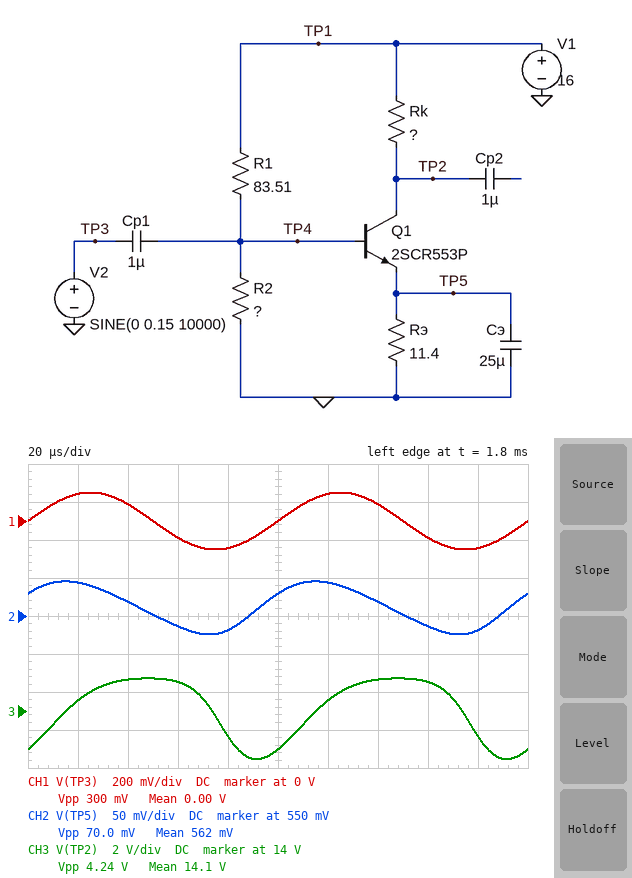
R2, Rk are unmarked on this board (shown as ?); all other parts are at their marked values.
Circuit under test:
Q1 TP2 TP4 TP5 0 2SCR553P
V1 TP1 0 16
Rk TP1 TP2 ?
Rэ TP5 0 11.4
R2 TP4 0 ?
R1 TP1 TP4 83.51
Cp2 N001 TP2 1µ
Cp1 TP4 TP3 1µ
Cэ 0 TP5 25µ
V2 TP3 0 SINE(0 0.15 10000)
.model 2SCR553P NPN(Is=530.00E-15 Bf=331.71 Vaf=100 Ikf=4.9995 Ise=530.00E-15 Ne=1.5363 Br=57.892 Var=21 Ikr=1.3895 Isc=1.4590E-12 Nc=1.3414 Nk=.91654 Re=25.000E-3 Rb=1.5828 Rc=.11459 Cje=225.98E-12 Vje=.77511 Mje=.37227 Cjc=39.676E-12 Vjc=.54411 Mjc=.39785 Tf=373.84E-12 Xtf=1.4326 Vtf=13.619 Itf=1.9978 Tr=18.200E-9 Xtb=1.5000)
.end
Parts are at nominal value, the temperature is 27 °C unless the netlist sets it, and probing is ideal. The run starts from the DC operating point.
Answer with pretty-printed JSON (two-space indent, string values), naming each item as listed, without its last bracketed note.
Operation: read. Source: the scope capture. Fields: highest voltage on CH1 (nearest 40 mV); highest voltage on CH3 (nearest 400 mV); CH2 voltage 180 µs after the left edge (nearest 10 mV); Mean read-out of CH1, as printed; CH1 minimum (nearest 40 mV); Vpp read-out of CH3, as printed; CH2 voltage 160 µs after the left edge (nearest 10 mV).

{
  "highest voltage on CH1": "160 mV",
  "highest voltage on CH3": "15.6 V",
  "CH2 voltage 180 µs after the left edge": "530 mV",
  "Mean read-out of CH1, as printed": "0.00 V",
  "CH1 minimum": "-160 mV",
  "Vpp read-out of CH3, as printed": "4.24 V",
  "CH2 voltage 160 µs after the left edge": "540 mV"
}
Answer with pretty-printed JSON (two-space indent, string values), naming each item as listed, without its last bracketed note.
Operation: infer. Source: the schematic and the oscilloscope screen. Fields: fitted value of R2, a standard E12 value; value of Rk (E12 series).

{
  "fitted value of R2, a standard E12 value": "6.8 Ω",
  "value of Rk": "39 Ω"
}
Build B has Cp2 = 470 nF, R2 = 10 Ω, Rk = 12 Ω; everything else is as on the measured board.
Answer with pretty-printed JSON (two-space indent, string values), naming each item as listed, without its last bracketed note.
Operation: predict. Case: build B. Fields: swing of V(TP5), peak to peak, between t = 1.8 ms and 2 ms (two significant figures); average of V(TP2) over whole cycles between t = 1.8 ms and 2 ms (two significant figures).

{
  "swing of V(TP5), peak to peak, between t = 1.8 ms and 2 ms": "120 mV",
  "average of V(TP2) over whole cycles between t = 1.8 ms and 2 ms": "15 V"
}
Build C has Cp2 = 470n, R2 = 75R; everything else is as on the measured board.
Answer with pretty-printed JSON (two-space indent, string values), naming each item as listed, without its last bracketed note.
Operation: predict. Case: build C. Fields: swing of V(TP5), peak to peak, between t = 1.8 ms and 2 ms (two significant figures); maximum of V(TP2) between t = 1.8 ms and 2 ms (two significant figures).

{
  "swing of V(TP5), peak to peak, between t = 1.8 ms and 2 ms": "11 mV",
  "maximum of V(TP2) between t = 1.8 ms and 2 ms": "4.2 V"
}
